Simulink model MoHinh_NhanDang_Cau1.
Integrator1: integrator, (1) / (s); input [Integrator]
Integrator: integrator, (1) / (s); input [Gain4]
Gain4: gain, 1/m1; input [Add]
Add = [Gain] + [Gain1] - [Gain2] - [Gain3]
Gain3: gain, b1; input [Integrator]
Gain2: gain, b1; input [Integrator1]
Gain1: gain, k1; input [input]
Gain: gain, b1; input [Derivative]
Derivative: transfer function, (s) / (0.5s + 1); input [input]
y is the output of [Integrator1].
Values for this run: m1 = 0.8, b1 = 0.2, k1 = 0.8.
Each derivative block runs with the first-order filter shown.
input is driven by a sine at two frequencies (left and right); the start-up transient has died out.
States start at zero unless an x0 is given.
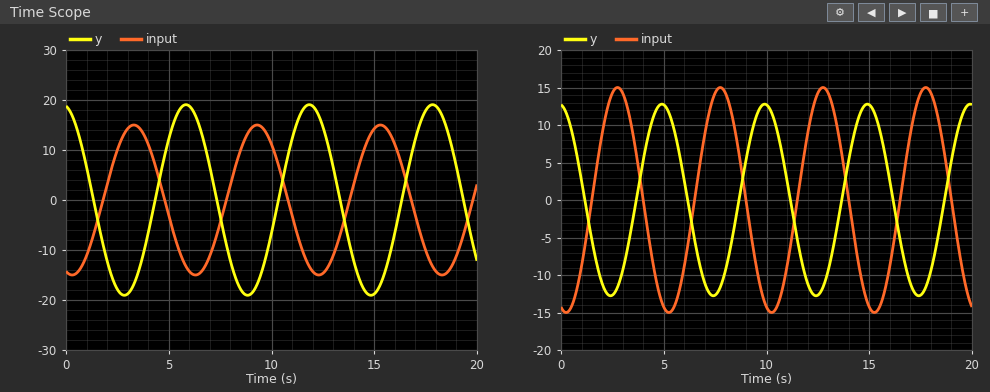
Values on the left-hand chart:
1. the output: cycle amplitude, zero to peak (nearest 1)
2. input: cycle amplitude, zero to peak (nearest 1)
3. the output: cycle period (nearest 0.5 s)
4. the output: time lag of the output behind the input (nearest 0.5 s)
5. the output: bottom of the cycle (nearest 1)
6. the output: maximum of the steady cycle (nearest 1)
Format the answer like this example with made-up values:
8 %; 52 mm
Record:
19; 15; 6.0 s; 2.5 s; -19; 19
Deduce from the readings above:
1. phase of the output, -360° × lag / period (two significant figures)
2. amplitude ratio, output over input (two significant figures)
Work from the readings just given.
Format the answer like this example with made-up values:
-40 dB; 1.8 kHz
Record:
-150°; 1.3
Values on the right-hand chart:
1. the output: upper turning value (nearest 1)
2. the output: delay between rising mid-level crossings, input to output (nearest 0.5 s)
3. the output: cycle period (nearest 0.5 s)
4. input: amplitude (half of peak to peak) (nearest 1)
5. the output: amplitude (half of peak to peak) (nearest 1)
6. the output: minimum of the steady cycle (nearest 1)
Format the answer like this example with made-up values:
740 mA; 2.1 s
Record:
13; 2.0 s; 5.0 s; 15; 13; -13
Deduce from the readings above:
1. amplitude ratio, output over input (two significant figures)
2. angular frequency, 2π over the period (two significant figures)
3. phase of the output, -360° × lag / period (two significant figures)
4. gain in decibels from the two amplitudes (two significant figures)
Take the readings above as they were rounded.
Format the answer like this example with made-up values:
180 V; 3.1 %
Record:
0.87; 1.3 rad/s; -140°; -1.2 dB
